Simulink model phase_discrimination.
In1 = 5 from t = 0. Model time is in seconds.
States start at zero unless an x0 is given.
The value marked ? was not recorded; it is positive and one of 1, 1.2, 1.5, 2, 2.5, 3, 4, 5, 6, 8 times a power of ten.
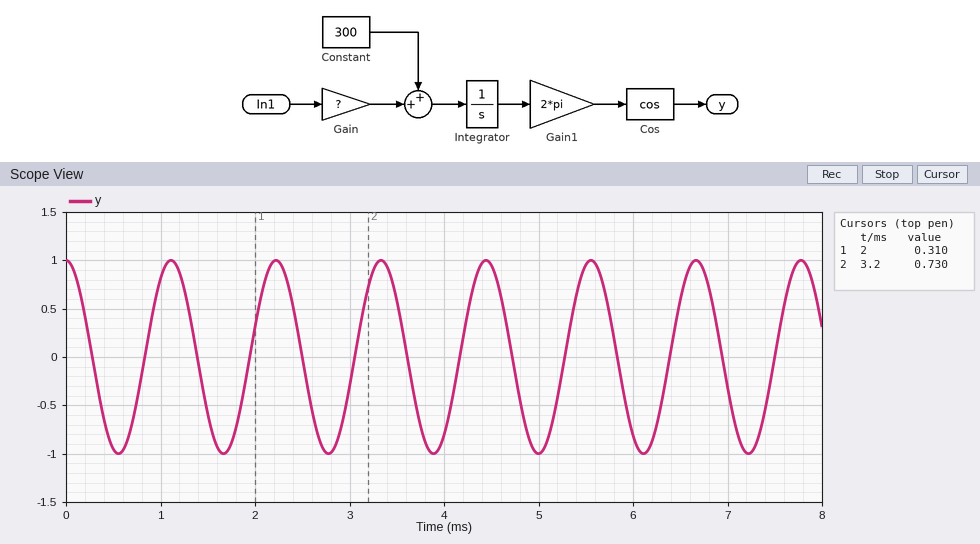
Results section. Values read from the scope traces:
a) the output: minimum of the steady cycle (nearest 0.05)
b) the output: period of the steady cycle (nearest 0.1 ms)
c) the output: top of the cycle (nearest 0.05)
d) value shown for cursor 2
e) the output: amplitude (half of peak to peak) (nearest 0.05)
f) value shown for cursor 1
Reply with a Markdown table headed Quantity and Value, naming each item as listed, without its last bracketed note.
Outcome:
| Quantity | Value |
|---|---|
| the output: minimum of the steady cycle | -1.00 |
| the output: period of the steady cycle | 1.1 ms |
| the output: top of the cycle | 1.00 |
| value shown for cursor 2 | 0.730 |
| the output: amplitude (half of peak to peak) | 1.00 |
| value shown for cursor 1 | 0.310 |
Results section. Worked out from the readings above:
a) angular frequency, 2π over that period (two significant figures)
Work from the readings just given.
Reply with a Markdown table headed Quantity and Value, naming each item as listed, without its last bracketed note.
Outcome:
| Quantity | Value |
|---|---|
| angular frequency, 2π over that period | 5.7 rad/ms |
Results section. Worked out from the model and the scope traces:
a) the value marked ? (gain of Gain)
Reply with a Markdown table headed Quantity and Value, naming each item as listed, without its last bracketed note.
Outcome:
| Quantity | Value |
|---|---|
| the value marked ? | 120 |
